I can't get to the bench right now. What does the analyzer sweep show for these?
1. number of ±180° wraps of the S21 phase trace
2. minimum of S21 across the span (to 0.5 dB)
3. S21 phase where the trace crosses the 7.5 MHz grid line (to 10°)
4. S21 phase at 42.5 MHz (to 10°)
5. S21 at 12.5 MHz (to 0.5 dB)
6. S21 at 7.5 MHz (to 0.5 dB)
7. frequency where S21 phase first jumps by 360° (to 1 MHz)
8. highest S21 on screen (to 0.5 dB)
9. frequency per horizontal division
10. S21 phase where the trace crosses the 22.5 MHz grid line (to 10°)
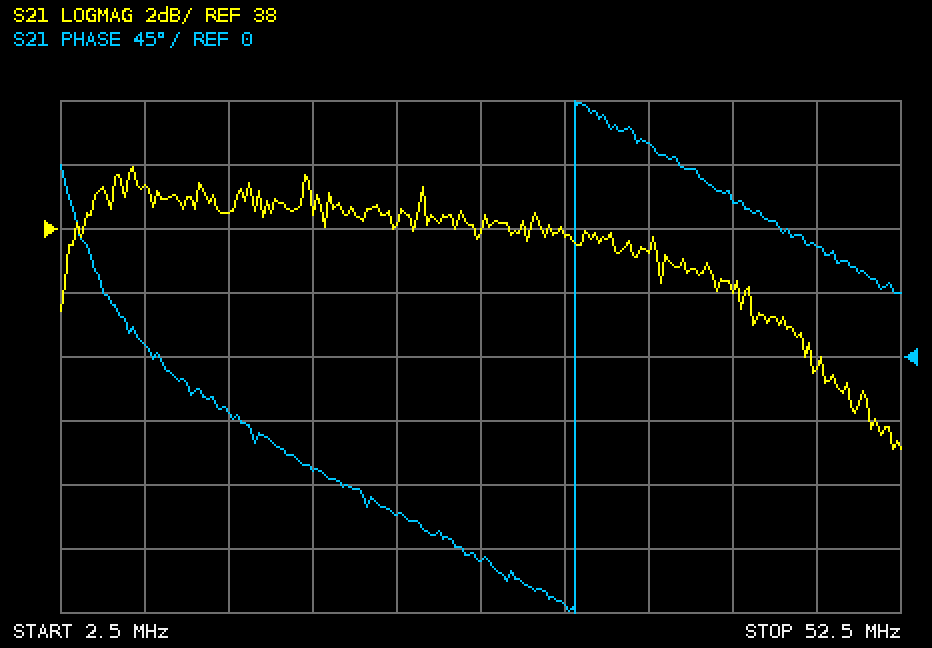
1
31.0 dB
10°
110°
38.5 dB
39.5 dB
33 MHz
40.0 dB
5 MHz
-110°
